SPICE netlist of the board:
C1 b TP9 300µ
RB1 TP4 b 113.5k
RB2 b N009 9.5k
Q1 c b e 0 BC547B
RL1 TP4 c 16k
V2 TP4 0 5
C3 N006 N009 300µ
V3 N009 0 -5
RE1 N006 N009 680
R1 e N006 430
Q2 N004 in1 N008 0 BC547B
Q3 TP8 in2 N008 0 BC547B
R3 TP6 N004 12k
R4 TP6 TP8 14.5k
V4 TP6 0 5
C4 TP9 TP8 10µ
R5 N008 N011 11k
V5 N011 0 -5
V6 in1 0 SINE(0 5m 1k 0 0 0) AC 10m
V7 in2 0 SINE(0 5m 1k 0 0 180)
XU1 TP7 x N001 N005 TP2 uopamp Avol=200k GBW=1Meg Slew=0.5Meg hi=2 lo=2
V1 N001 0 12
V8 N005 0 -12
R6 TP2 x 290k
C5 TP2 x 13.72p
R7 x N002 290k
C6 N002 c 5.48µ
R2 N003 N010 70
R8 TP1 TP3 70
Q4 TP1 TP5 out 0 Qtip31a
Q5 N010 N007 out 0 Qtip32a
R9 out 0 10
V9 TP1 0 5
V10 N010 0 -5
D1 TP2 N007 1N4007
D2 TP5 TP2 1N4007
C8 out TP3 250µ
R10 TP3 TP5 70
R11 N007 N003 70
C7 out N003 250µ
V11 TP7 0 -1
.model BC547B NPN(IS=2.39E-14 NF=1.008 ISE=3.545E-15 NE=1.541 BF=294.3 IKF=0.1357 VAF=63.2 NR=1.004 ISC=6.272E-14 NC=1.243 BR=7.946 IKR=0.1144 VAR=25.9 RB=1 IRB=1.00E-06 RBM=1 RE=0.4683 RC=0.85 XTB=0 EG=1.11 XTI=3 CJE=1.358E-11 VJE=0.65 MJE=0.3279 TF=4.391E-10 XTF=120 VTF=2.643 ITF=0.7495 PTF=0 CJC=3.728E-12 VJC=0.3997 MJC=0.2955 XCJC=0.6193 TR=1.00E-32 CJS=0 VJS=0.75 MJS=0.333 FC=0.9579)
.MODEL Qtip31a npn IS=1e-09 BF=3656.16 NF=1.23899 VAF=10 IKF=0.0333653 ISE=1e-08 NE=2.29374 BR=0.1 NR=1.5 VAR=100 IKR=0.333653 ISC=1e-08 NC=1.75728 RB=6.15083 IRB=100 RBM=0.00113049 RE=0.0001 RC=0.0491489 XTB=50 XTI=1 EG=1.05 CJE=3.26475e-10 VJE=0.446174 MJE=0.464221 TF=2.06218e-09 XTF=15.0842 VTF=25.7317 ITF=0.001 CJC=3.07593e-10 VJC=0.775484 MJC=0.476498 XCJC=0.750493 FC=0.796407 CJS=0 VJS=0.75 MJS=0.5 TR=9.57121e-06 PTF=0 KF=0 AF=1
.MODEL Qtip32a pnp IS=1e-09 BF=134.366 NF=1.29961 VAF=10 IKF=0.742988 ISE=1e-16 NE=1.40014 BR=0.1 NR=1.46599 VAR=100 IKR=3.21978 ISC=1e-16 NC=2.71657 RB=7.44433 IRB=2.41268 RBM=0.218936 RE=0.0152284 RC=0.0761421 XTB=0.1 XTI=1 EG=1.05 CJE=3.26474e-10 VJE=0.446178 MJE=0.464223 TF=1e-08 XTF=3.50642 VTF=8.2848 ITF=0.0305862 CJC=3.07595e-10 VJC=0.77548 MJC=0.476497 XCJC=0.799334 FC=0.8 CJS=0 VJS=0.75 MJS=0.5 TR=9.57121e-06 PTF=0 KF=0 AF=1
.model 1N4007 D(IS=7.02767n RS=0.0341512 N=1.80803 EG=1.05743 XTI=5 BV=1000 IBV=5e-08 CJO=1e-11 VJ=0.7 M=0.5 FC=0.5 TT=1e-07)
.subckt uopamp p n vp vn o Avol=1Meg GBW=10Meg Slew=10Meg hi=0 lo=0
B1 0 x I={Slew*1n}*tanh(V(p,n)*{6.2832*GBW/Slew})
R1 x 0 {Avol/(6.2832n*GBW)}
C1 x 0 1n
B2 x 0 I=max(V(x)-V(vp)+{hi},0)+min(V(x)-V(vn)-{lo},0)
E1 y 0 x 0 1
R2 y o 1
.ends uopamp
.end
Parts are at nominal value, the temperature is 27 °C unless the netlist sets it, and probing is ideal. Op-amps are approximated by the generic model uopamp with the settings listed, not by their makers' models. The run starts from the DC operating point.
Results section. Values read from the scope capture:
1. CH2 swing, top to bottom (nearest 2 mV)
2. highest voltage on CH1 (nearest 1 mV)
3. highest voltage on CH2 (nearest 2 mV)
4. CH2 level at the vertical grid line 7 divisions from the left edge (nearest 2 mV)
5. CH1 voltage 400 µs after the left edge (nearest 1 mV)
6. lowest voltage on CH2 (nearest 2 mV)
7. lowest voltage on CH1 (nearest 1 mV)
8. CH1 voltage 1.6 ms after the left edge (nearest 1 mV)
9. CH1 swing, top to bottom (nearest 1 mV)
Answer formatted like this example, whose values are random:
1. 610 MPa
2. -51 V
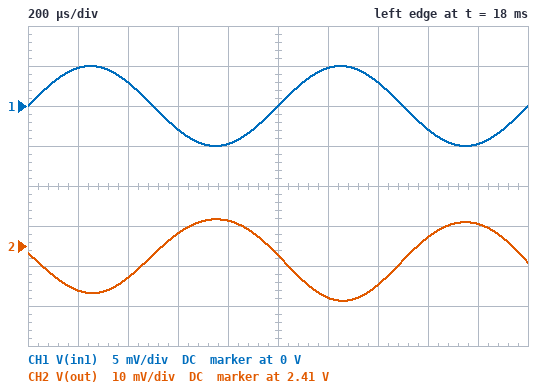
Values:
1. 20 mV
2. 5 mV
3. 2.416 V
4. 2.400 V
5. 3 mV
6. 2.396 V
7. -5 mV
8. -3 mV
9. 10 mV
